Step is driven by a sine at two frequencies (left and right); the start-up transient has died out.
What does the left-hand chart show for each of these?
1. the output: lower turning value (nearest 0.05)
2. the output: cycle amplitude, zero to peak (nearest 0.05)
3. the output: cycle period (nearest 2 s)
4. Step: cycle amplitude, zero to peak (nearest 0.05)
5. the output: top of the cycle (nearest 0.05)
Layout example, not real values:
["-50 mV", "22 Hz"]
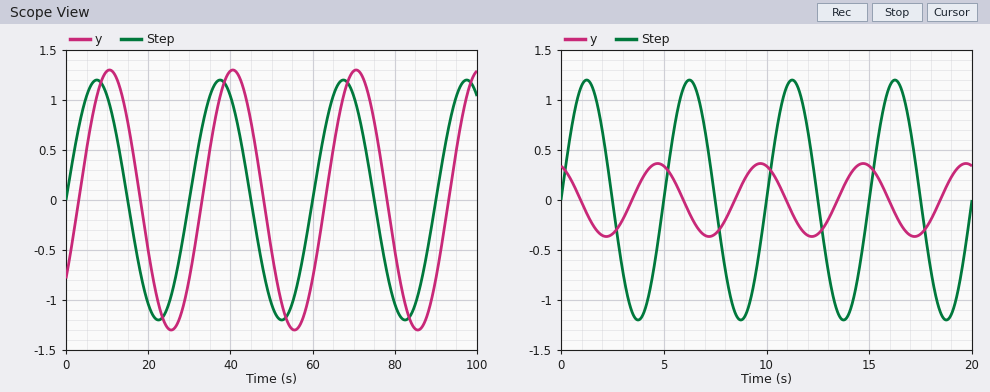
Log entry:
["-1.30", "1.30", "30 s", "1.20", "1.30"]
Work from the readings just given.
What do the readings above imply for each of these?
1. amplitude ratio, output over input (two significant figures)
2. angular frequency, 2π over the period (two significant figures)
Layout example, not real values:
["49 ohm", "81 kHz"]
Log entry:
["1.1", "0.21 rad/s"]
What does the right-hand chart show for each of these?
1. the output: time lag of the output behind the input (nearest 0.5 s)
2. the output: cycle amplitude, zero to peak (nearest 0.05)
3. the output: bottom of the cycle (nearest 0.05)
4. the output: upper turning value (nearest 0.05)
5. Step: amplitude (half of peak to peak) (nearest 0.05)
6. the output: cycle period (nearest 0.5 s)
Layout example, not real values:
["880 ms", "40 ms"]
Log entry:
["3.5 s", "0.35", "-0.35", "0.35", "1.20", "5.0 s"]
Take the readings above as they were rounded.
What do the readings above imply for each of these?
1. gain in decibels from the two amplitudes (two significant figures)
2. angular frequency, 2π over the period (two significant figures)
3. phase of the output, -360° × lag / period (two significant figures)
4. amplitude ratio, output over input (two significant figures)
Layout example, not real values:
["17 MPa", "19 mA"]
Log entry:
["-11 dB", "1.3 rad/s", "-250°", "0.29"]
